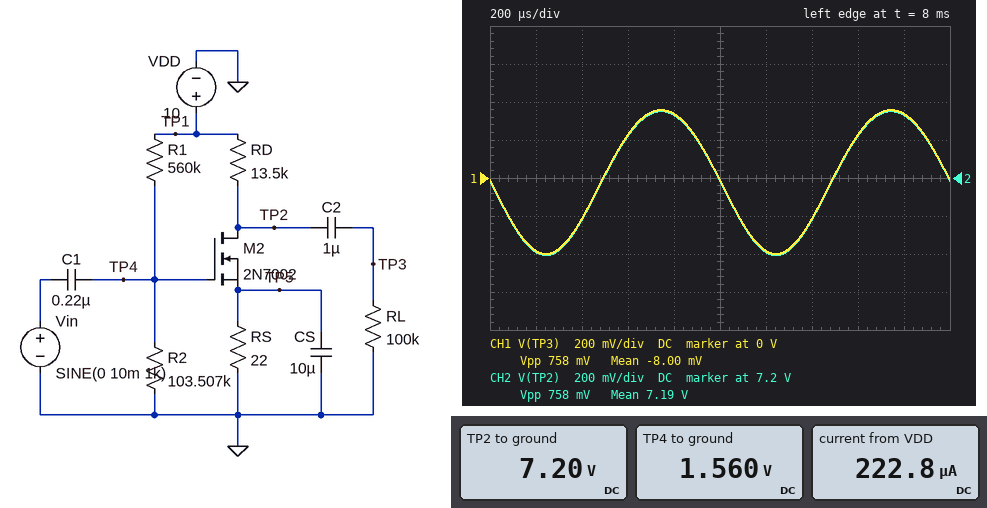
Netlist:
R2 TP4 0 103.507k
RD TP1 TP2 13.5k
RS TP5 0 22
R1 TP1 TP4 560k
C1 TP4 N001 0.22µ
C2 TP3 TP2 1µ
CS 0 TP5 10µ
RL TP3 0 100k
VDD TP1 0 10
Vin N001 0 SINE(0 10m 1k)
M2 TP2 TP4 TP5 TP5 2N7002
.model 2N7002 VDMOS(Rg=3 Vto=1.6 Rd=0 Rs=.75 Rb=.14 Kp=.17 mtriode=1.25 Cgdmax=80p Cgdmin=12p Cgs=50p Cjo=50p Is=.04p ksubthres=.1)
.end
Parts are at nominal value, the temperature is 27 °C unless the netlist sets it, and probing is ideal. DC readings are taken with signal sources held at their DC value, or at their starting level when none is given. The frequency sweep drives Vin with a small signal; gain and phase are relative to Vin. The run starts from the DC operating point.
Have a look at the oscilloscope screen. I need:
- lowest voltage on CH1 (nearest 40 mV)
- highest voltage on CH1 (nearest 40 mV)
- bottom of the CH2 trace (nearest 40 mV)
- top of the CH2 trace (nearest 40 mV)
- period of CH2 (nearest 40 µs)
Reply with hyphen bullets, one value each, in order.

- -400 mV
- 360 mV
- 6.80 V
- 7.56 V
- 1.00 ms
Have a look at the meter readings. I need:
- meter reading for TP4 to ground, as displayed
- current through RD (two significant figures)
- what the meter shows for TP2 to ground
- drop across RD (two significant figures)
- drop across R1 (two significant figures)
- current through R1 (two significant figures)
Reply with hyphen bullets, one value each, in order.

- 1.560 V
- 210 µA
- 7.20 V
- 2.8 V
- 8.4 V
- 15 µA
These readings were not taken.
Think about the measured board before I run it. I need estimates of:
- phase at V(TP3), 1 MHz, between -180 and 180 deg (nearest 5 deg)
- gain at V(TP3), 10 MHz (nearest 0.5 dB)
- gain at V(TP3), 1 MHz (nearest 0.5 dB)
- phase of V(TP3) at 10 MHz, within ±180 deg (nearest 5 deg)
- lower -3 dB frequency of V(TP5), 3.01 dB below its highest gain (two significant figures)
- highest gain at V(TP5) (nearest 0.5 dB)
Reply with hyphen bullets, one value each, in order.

- 110 deg
- 4.5 dB
- 23.5 dB
- 75 deg
- 8.1 Hz
- -23.5 dB
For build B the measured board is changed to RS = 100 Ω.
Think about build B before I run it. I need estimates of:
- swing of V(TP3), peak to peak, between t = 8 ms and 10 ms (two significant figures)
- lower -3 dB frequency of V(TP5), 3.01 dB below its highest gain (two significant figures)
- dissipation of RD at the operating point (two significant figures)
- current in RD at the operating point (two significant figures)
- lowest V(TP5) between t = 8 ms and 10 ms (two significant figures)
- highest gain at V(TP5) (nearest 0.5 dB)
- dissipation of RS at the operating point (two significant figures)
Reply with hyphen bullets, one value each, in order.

- 650 mV
- 7.7 Hz
- 390 µW
- 170 µA
- 17 mV
- -13.5 dB
- 2.9 µW
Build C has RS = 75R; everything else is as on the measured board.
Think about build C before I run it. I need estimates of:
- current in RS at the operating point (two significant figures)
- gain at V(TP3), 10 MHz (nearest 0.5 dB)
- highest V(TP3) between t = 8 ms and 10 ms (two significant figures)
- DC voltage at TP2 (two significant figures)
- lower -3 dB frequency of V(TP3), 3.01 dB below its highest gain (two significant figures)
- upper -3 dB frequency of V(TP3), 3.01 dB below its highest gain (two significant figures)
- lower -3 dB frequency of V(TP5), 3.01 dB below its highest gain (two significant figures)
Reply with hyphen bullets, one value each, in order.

- 180 µA
- 3.5 dB
- 320 mV
- 7.6 V
- 14 Hz
- 420 kHz
- 7.8 Hz
